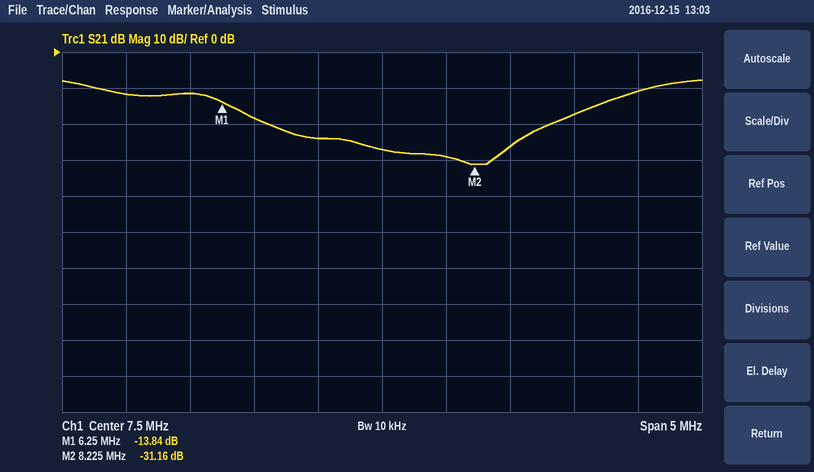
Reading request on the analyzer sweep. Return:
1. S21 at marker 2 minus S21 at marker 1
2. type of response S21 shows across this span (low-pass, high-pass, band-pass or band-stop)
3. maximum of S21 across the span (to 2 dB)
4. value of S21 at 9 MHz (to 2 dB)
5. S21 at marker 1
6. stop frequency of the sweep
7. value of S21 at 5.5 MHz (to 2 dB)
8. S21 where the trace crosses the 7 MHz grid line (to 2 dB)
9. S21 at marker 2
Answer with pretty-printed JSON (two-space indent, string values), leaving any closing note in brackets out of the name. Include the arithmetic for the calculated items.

{
  "S21 at marker 2 minus S21 at marker 1": "-31.16 − (-13.84) = -17.32 dB",
  "type of response S21 shows across this span": "band-stop",
  "maximum of S21 across the span": "-8 dB",
  "value of S21 at 9 MHz": "-18 dB",
  "S21 at marker 1": "-13.84 dB",
  "stop frequency of the sweep": "10 MHz",
  "value of S21 at 5.5 MHz": "-12 dB",
  "S21 where the trace crosses the 7 MHz grid line": "-24 dB",
  "S21 at marker 2": "-31.16 dB"
}
